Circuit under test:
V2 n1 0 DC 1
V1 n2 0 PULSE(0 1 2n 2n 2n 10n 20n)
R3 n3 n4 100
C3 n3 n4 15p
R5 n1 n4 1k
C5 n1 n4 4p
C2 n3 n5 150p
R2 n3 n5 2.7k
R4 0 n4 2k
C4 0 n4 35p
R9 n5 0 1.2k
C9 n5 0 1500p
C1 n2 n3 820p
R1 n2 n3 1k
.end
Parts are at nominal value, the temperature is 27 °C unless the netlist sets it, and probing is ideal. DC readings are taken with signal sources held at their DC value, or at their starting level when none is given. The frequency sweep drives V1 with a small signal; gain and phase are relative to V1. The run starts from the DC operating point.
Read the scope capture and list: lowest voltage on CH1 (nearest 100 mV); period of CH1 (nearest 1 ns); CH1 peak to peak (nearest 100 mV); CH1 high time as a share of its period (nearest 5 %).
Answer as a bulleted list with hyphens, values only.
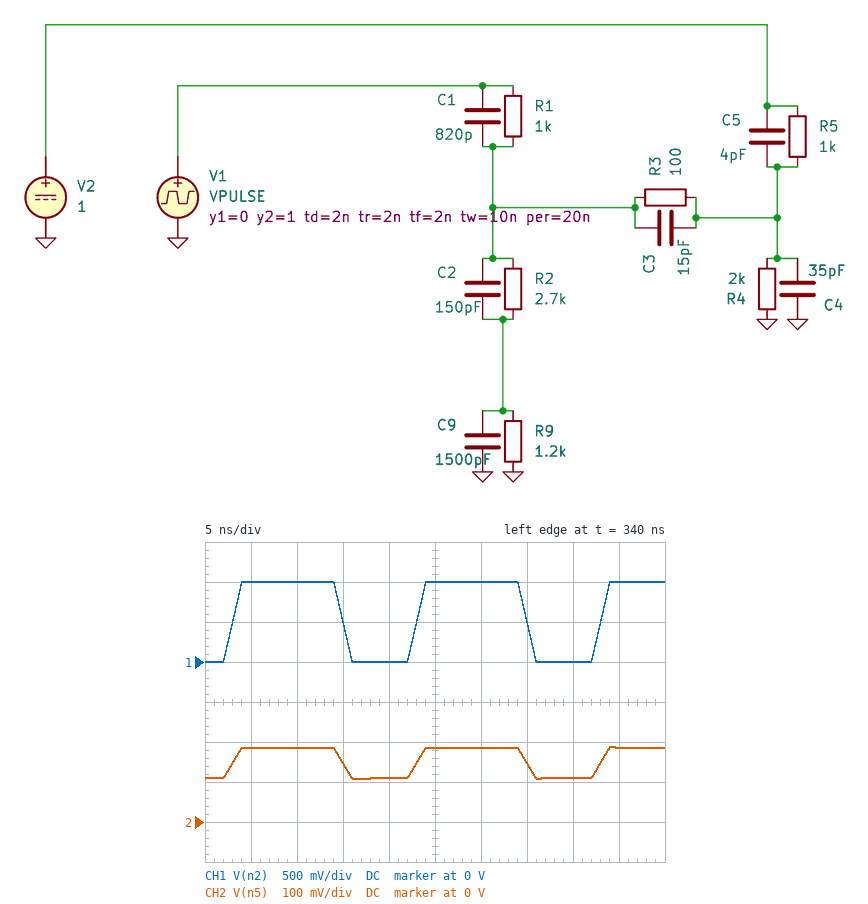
- 0 V
- 20 ns
- 1.0 V
- 60 %
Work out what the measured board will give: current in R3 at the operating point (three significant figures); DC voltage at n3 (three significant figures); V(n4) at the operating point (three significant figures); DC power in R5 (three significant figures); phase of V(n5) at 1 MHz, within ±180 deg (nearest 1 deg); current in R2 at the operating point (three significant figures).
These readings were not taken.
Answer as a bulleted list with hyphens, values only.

- 427 µA
- 340 mV
- 382 mV
- 382 µW
- -3 deg
- 87.1 µA
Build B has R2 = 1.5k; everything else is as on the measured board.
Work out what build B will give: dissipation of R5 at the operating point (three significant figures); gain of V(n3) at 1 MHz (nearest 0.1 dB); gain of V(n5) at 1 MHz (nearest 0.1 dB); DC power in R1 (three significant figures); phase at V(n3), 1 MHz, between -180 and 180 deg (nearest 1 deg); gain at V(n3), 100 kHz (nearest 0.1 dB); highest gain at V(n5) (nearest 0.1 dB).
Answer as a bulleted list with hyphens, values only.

- 397 µW
- -2.3 dB
- -21.5 dB
- 106 µW
- 14 deg
- -8.0 dB
- -15.6 dB
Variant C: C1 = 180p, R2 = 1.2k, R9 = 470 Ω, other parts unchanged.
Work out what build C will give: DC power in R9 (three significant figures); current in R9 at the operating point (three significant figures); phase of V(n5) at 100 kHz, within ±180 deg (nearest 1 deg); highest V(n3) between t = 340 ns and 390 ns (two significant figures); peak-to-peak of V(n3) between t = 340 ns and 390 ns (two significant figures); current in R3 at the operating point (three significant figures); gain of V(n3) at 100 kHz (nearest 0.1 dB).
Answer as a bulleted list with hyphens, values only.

- 15.1 µW
- 179 µA
- -11 deg
- 740 mV
- 570 mV
- 479 µA
- -9.3 dB
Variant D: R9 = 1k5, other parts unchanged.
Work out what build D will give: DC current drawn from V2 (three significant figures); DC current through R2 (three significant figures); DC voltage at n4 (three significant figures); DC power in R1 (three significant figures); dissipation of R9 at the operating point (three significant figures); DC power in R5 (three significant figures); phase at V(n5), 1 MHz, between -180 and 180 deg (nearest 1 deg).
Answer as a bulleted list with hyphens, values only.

- 616 µA
- 81.4 µA
- 384 mV
- 117 µW
- 9.95 µW
- 379 µW
- -4 deg
